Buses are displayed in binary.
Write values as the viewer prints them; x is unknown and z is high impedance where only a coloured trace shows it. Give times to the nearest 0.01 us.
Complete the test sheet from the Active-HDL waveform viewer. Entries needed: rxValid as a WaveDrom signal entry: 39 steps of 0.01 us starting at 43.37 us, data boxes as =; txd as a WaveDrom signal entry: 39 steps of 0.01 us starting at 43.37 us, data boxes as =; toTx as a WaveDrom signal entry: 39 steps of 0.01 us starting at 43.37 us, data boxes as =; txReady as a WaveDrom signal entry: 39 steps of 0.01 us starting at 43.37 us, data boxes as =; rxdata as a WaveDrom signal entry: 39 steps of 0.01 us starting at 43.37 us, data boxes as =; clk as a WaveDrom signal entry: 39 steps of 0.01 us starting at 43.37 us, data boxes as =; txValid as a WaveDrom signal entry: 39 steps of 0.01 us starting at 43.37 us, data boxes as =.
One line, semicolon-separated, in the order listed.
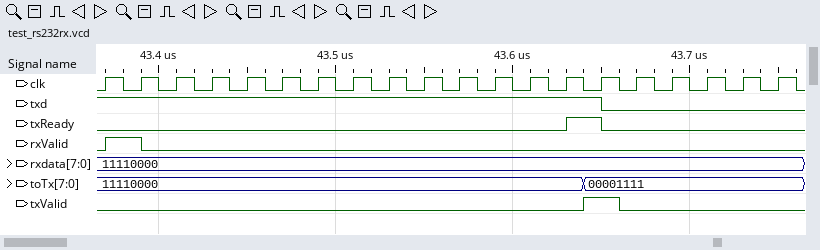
{name: 'rxValid', wave: '1.0....................................'}; {name: 'txd', wave: '1...........................0..........'}; {name: 'toTx', wave: '=..........................=...........', data: '11110000 00001111'}; {name: 'txReady', wave: '0.........................1.0..........'}; {name: 'rxdata', wave: '=......................................', data: '11110000'}; {name: 'clk', wave: '101010101010101010101010101010101010101'}; {name: 'txValid', wave: '0..........................1.0.........'}
